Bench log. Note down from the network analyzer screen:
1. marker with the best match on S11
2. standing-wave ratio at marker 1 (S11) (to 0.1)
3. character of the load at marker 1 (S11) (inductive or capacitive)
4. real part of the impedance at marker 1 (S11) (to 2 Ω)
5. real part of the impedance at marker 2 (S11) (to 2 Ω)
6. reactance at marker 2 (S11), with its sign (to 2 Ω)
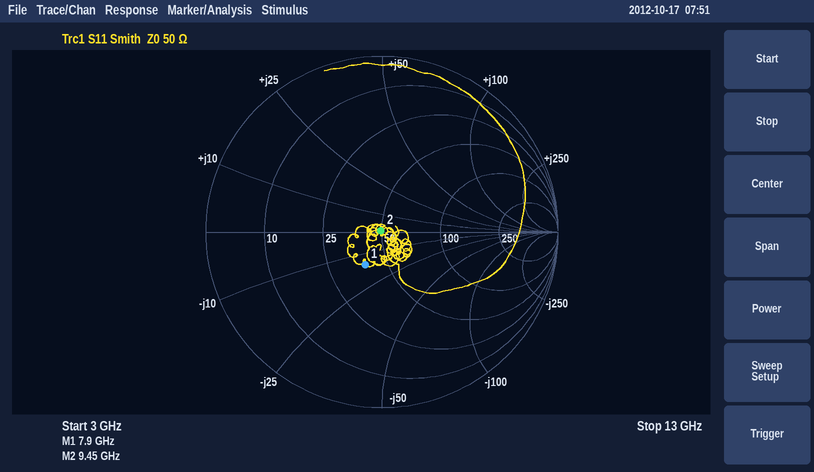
marker 2
1.5
capacitive
38 Ω
50 Ω
0 Ω
